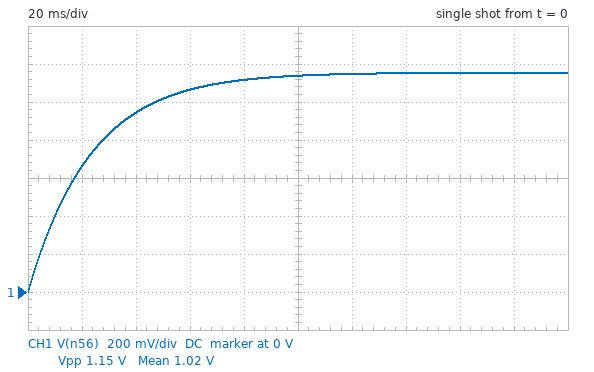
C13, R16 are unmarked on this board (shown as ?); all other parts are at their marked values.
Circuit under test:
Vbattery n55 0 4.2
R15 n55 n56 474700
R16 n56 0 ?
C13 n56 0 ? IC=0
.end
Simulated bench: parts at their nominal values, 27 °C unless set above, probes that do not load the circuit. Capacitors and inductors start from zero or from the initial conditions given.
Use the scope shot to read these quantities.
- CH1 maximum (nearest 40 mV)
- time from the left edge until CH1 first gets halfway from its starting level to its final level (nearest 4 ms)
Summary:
1.16 V
16 ms
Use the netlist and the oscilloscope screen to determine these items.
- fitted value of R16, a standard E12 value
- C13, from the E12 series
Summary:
180 kΩ
180 nF
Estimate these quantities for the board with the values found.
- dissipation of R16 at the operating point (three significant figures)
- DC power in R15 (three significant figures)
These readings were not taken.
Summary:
7.41 µW
19.5 µW
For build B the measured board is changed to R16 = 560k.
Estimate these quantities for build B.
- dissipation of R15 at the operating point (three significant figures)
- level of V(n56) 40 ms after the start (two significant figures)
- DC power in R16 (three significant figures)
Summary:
7.82 µW
1.3 V
9.23 µW
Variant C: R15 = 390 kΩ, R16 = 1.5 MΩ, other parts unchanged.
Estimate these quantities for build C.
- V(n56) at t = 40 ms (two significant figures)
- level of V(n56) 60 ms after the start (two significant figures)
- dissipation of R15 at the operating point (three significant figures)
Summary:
1.7 V
2.2 V
1.93 µW
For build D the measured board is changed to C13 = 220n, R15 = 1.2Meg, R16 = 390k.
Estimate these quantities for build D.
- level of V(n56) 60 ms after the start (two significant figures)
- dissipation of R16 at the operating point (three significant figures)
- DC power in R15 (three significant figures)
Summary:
620 mV
2.72 µW
8.37 µW
